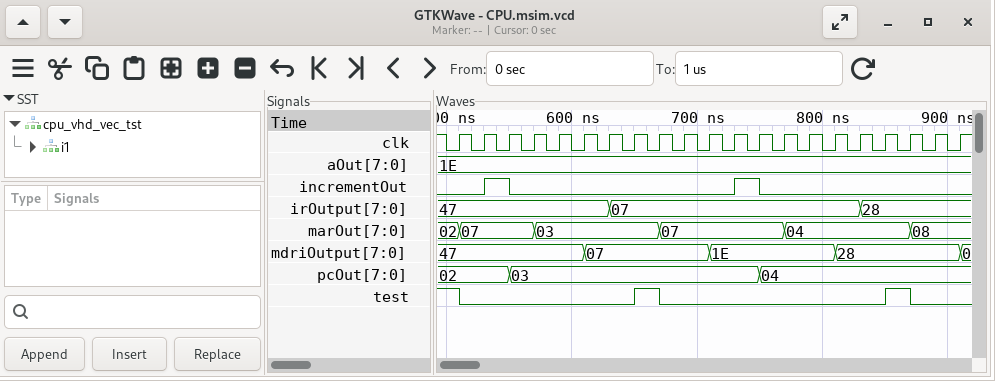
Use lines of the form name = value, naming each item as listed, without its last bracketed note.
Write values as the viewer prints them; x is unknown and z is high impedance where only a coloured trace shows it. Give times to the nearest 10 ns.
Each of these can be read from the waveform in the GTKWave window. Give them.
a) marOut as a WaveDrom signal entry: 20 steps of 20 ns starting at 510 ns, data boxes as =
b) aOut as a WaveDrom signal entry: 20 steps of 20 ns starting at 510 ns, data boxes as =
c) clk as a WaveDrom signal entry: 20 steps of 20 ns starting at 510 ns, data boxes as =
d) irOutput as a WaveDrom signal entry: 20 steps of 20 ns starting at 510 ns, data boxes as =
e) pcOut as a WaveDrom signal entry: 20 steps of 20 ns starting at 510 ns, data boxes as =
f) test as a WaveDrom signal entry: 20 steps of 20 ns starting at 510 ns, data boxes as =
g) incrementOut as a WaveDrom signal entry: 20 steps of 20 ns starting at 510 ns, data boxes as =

marOut as a WaveDrom signal entry: 20 steps of 20 ns starting at 510 ns, data boxes as = = {name: 'marOut', wave: '=..=....=....=....=.', data: '07 03 07 04 08'}
aOut as a WaveDrom signal entry: 20 steps of 20 ns starting at 510 ns, data boxes as = = {name: 'aOut', wave: '=...................', data: '1E'}
clk as a WaveDrom signal entry: 20 steps of 20 ns starting at 510 ns, data boxes as = = {name: 'clk', wave: 'p...................'}
irOutput as a WaveDrom signal entry: 20 steps of 20 ns starting at 510 ns, data boxes as = = {name: 'irOutput', wave: '=.....=.........=...', data: '47 07 28'}
pcOut as a WaveDrom signal entry: 20 steps of 20 ns starting at 510 ns, data boxes as = = {name: 'pcOut', wave: '=.=.........=.......', data: '02 03 04'}
test as a WaveDrom signal entry: 20 steps of 20 ns starting at 510 ns, data boxes as = = {name: 'test', wave: '0......10........10.'}
incrementOut as a WaveDrom signal entry: 20 steps of 20 ns starting at 510 ns, data boxes as = = {name: 'incrementOut', wave: '010........10.......'}
